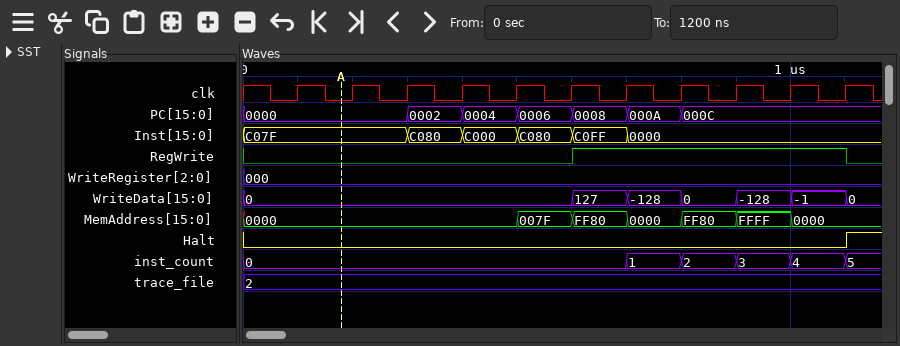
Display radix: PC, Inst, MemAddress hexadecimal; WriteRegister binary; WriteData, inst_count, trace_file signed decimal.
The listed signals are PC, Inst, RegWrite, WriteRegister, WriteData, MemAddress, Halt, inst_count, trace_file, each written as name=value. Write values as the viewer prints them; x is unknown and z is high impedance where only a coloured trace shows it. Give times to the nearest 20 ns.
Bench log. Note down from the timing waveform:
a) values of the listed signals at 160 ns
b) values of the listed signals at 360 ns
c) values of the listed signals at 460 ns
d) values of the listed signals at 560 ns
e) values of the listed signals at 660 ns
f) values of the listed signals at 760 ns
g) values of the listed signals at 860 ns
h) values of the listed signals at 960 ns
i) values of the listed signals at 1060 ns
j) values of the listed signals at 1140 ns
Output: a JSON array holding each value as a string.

["PC=0000, Inst=C07F, RegWrite=0, WriteRegister=000, WriteData=0, MemAddress=0000, Halt=0, inst_count=0, trace_file=2", "PC=0002, Inst=C080, RegWrite=0, WriteRegister=000, WriteData=0, MemAddress=0000, Halt=0, inst_count=0, trace_file=2", "PC=0004, Inst=C000, RegWrite=0, WriteRegister=000, WriteData=0, MemAddress=0000, Halt=0, inst_count=0, trace_file=2", "PC=0006, Inst=C080, RegWrite=0, WriteRegister=000, WriteData=0, MemAddress=007F, Halt=0, inst_count=0, trace_file=2", "PC=0008, Inst=C0FF, RegWrite=1, WriteRegister=000, WriteData=127, MemAddress=FF80, Halt=0, inst_count=0, trace_file=2", "PC=000A, Inst=0000, RegWrite=1, WriteRegister=000, WriteData=-128, MemAddress=0000, Halt=0, inst_count=1, trace_file=2", "PC=000C, Inst=0000, RegWrite=1, WriteRegister=000, WriteData=0, MemAddress=FF80, Halt=0, inst_count=2, trace_file=2", "PC=000C, Inst=0000, RegWrite=1, WriteRegister=000, WriteData=-128, MemAddress=FFFF, Halt=0, inst_count=3, trace_file=2", "PC=000C, Inst=0000, RegWrite=1, WriteRegister=000, WriteData=-1, MemAddress=0000, Halt=0, inst_count=4, trace_file=2", "PC=000C, Inst=0000, RegWrite=0, WriteRegister=000, WriteData=0, MemAddress=0000, Halt=1, inst_count=5, trace_file=2"]
